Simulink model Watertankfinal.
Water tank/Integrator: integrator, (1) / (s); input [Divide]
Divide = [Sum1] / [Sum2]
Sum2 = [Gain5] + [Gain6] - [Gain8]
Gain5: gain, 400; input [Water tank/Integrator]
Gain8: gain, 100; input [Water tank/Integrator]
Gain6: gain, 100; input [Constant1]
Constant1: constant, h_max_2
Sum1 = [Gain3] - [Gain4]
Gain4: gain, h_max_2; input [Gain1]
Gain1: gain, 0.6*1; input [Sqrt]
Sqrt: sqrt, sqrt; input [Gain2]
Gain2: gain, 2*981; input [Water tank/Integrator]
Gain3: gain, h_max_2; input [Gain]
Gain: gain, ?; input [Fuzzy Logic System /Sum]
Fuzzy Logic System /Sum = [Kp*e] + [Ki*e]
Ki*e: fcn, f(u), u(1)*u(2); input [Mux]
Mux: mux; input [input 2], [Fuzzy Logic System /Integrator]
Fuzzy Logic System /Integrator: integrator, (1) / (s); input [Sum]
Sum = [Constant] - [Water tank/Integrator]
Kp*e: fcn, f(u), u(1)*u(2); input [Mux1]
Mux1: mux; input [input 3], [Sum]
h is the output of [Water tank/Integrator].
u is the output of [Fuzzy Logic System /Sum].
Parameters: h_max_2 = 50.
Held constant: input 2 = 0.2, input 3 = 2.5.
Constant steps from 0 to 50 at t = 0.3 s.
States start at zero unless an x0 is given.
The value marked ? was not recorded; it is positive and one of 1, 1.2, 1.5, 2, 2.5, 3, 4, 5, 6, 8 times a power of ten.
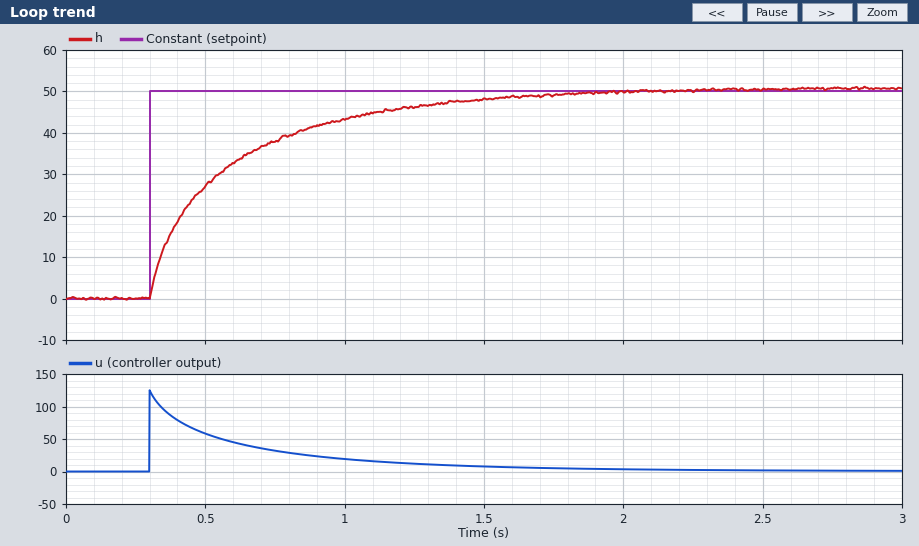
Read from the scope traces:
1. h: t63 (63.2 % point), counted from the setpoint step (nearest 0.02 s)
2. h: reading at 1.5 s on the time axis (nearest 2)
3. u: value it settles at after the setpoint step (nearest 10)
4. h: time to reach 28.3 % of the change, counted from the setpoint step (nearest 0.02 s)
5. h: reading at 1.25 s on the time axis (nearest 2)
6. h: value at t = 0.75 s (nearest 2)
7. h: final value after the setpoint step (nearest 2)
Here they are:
0.28 s
48
0
0.06 s
46
38
50
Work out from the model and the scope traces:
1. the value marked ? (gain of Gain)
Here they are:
300
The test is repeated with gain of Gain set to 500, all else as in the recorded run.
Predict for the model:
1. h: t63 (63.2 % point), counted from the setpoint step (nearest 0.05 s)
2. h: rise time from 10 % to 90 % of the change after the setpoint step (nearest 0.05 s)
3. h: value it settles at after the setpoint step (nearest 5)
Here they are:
0.15 s
0.50 s
50
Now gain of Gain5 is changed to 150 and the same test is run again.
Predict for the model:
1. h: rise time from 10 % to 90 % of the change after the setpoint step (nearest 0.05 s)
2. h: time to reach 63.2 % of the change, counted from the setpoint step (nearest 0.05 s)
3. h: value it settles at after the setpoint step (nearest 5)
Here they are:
0.40 s
0.15 s
50
